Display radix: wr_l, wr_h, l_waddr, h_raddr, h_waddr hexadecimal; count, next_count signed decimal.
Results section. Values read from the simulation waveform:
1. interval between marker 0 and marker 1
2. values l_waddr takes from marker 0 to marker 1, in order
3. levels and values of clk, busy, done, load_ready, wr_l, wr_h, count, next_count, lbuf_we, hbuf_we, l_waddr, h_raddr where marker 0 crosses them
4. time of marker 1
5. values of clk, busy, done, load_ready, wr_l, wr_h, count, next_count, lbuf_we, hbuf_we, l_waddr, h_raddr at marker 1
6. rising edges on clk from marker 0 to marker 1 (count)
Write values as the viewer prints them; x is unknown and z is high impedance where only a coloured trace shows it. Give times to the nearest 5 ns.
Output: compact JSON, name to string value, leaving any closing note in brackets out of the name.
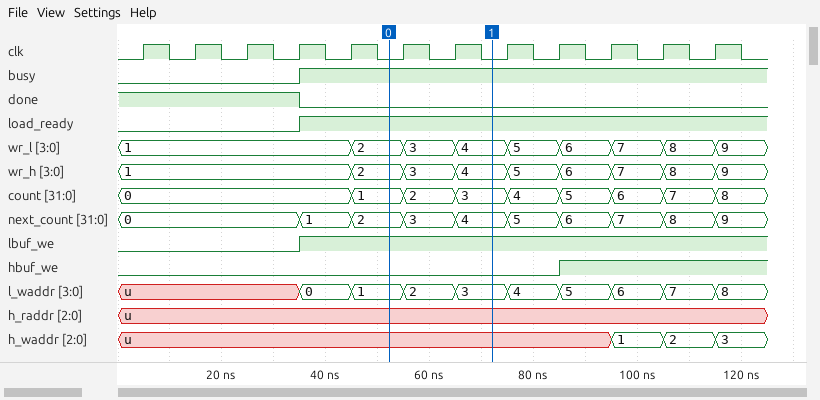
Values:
{"interval between marker 0 and marker 1": "20 ns", "values l_waddr takes from marker 0 to marker 1, in order": "1, 2, 3", "levels and values of clk, busy, done, load_ready, wr_l, wr_h, count, next_count, lbuf_we, hbuf_we, l_waddr, h_raddr where marker 0 crosses them": "clk=0, busy=1, done=0, load_ready=1, wr_l=2, wr_h=2, count=1, next_count=2, lbuf_we=1, hbuf_we=0, l_waddr=1, h_raddr=u", "time of marker 1": "70 ns", "values of clk, busy, done, load_ready, wr_l, wr_h, count, next_count, lbuf_we, hbuf_we, l_waddr, h_raddr at marker 1": "clk=0, busy=1, done=0, load_ready=1, wr_l=4, wr_h=4, count=3, next_count=4, lbuf_we=1, hbuf_we=0, l_waddr=3, h_raddr=u", "rising edges on clk from marker 0 to marker 1": "2"}
